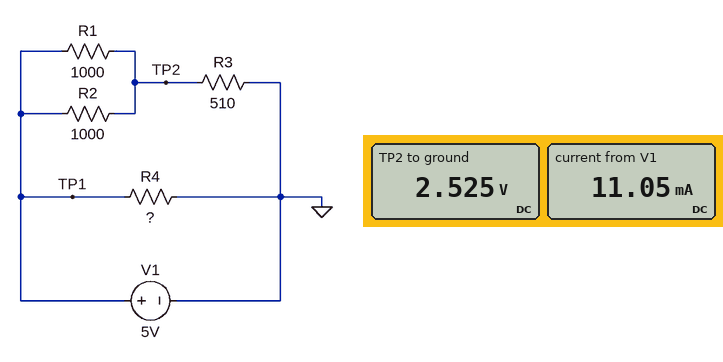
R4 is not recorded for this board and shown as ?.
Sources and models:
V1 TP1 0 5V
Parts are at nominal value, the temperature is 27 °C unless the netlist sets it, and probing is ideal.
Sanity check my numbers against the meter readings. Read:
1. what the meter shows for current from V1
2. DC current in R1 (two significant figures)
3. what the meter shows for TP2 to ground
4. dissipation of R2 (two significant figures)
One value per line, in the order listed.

11.05 mA
2.5 mA
2.525 V
6.1 mW
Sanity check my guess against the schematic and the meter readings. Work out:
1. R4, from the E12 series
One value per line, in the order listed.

820 Ω
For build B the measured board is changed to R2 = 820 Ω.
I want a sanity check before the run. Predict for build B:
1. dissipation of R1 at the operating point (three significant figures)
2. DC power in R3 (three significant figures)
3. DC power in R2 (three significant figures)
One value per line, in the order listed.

5.50 mW
13.8 mW
6.71 mW
